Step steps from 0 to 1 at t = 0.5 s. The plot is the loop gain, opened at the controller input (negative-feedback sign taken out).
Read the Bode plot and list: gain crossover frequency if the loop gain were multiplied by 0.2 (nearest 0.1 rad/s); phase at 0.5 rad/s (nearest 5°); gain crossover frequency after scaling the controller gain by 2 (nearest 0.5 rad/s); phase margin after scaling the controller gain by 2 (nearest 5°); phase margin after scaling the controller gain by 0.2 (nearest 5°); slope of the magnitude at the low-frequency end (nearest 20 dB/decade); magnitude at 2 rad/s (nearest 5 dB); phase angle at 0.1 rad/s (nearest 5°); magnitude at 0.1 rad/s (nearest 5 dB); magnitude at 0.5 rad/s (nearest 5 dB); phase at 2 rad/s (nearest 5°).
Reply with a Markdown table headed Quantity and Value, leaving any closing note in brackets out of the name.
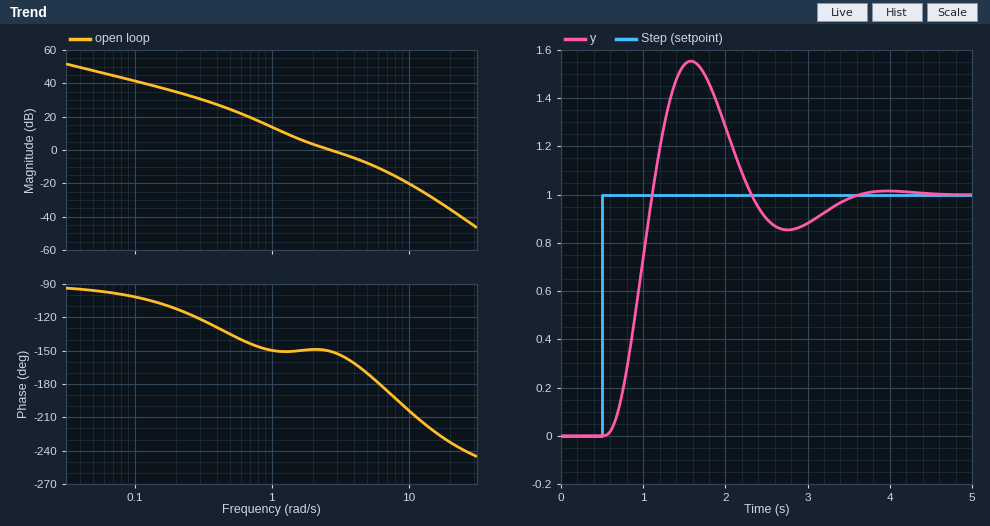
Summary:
| Quantity | Value |
|---|---|
| gain crossover frequency if the loop gain were multiplied by 0.2 | 1.0 rad/s |
| phase at 0.5 rad/s | -135° |
| gain crossover frequency after scaling the controller gain by 2 | 4.5 rad/s |
| phase margin after scaling the controller gain by 2 | 15° |
| phase margin after scaling the controller gain by 0.2 | 30° |
| slope of the magnitude at the low-frequency end | -20 dB/decade |
| magnitude at 2 rad/s | 5 dB |
| phase angle at 0.1 rad/s | -100° |
| magnitude at 0.1 rad/s | 40 dB |
| magnitude at 0.5 rad/s | 25 dB |
| phase at 2 rad/s | -150° |
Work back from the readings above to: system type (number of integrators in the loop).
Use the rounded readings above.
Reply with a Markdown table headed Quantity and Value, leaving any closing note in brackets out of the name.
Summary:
| Quantity | Value |
|---|---|
| system type | 1 |
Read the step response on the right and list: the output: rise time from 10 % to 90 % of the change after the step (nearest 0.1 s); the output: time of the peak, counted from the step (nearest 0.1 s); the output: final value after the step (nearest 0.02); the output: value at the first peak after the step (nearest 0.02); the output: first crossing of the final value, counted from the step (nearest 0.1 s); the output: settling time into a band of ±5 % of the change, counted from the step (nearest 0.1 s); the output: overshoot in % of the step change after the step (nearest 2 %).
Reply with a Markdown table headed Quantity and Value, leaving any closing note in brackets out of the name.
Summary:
| Quantity | Value |
|---|---|
| the output: rise time from 10 % to 90 % of the change after the step | 0.4 s |
| the output: time of the peak, counted from the step | 1.1 s |
| the output: final value after the step | 1.00 |
| the output: value at the first peak after the step | 1.56 |
| the output: first crossing of the final value, counted from the step | 0.6 s |
| the output: settling time into a band of ±5 % of the change, counted from the step | 2.8 s |
| the output: overshoot in % of the step change after the step | 56 % |
